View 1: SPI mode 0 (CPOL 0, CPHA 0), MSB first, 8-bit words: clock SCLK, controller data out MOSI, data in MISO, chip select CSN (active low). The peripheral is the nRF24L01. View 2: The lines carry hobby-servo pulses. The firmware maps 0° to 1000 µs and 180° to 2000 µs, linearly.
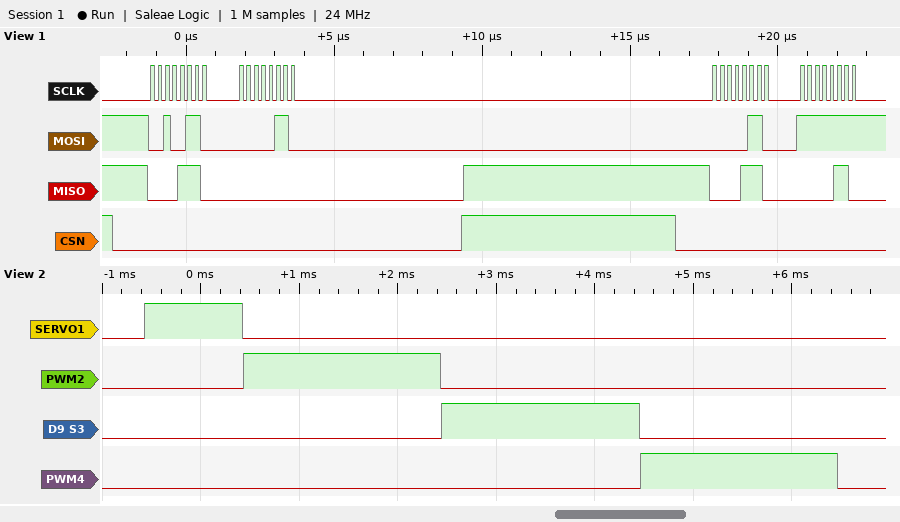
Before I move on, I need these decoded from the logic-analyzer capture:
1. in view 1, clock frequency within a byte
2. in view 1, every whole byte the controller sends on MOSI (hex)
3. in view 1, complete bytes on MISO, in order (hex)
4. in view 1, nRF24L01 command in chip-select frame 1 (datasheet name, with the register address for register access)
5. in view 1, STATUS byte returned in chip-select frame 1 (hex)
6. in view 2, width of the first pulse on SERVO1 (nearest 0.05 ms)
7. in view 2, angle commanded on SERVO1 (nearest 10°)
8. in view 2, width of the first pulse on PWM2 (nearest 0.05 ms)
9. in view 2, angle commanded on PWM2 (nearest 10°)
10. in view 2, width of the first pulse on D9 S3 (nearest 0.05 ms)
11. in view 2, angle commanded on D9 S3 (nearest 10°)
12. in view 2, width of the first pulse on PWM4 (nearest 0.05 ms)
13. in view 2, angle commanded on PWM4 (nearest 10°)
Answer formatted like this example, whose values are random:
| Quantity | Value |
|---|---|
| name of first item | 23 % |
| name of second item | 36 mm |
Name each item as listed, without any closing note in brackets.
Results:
| Quantity | Value |
|---|---|
| in view 1, clock frequency within a byte | 4 MHz |
| in view 1, every whole byte the controller sends on MOSI | 0x26 0x06 0x06 0xFF |
| in view 1, complete bytes on MISO, in order | 0x0E 0x00 0x0E 0x06 |
| in view 1, nRF24L01 command in chip-select frame 1 | W_REGISTER 0x06 |
| in view 1, STATUS byte returned in chip-select frame 1 | 0x0E |
| in view 2, width of the first pulse on SERVO1 | 1.00 ms |
| in view 2, angle commanded on SERVO1 | 0° |
| in view 2, width of the first pulse on PWM2 | 2.00 ms |
| in view 2, angle commanded on PWM2 | 180° |
| in view 2, width of the first pulse on D9 S3 | 2.00 ms |
| in view 2, angle commanded on D9 S3 | 180° |
| in view 2, width of the first pulse on PWM4 | 2.00 ms |
| in view 2, angle commanded on PWM4 | 180° |
